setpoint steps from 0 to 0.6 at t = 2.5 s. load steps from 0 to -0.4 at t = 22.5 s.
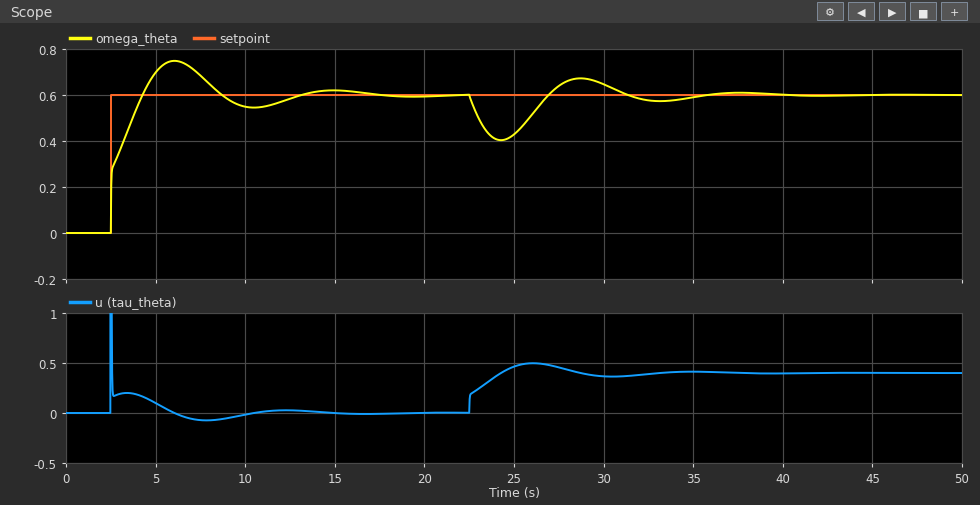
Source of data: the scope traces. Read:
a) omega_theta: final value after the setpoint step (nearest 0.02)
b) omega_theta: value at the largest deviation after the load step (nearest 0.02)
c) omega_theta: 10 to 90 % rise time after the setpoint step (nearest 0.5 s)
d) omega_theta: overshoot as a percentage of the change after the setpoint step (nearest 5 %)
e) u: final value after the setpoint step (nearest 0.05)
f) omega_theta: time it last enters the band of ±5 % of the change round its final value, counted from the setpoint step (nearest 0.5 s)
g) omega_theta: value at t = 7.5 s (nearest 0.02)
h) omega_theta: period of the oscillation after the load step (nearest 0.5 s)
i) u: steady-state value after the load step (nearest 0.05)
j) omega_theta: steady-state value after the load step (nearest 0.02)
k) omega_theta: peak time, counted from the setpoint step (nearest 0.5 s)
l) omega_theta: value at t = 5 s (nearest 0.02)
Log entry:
0.60
0.40
1.5 s
25 %
0.00
9.5 s
0.68
9.0 s
0.40
0.60
3.5 s
0.70
